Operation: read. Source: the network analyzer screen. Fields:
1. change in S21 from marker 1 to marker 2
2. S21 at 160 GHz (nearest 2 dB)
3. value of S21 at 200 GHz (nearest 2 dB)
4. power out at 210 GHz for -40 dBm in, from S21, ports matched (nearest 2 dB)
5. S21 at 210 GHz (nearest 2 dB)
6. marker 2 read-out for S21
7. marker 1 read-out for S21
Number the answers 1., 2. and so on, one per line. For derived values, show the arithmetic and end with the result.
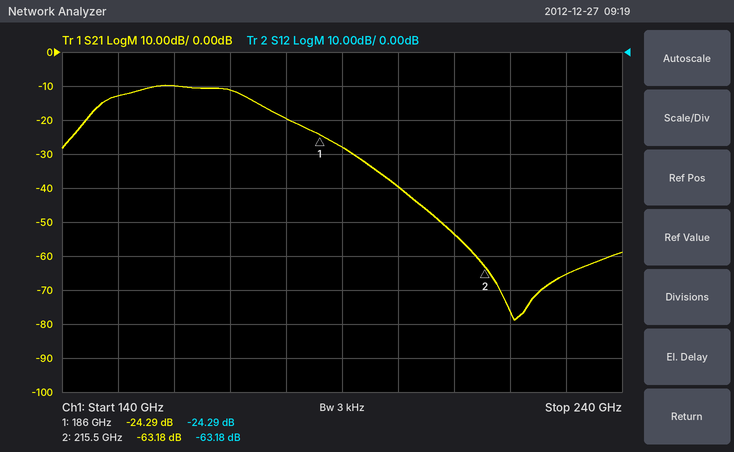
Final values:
1. -63.18 − (-24.29) = -38.89 dB
2. -10 dB
3. -40 dB
4. -40 dBm + (-54 dB) = -94 dBm
5. -54 dB
6. -63.18 dB
7. -24.29 dB
